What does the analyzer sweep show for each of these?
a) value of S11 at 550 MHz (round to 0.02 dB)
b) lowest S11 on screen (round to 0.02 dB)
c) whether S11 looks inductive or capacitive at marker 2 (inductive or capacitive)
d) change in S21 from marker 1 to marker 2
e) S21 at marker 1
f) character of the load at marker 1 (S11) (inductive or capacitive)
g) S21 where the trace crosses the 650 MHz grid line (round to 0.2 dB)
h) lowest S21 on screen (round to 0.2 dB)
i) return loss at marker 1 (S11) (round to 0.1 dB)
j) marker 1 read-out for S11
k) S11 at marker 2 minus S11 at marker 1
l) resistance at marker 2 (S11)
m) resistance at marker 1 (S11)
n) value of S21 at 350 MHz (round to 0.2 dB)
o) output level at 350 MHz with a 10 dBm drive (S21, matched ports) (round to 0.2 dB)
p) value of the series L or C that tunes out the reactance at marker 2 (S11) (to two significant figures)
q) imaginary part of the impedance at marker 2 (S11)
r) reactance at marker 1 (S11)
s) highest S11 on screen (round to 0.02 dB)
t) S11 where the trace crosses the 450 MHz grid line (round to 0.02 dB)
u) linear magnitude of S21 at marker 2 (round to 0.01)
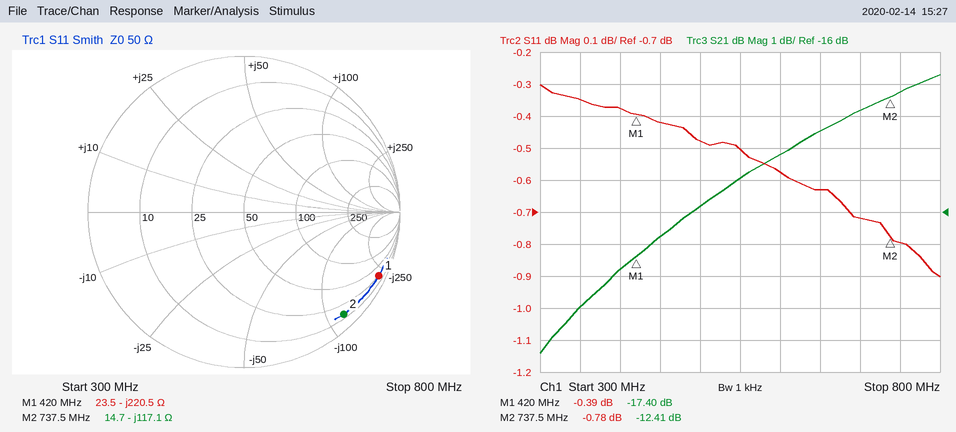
-0.50 dB
-0.90 dB
capacitive
4.99 dB
-17.40 dB
capacitive
-13.4 dB
-20.4 dB
0.4 dB
-0.39 dB
-0.39 dB
14.7 Ω
23.5 Ω
-19.0 dB
-9.0 dBm
25 nH
-117.1 Ω
-220.5 Ω
-0.30 dB
-0.42 dB
0.24
